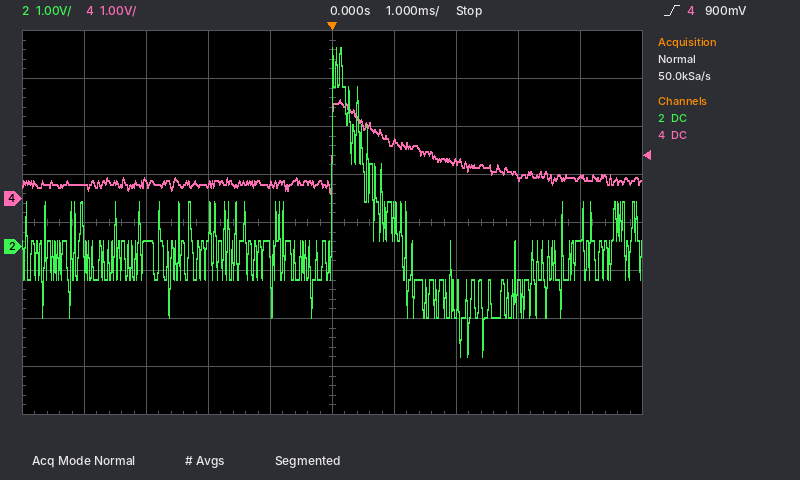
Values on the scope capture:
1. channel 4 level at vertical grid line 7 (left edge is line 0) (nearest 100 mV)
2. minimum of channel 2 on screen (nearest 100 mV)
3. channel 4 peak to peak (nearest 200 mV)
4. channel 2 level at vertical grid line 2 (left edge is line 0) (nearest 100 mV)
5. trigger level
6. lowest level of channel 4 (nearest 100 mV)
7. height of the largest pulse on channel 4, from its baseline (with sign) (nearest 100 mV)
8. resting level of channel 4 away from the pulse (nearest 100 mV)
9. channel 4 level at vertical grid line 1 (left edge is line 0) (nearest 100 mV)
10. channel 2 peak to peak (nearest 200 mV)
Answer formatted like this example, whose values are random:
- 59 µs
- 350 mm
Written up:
- 800 mV
- -2.3 V
- 2.0 V
- 100 mV
- 900 mV
- 100 mV
- +1.7 V
- 300 mV
- 300 mV
- 6.4 V
